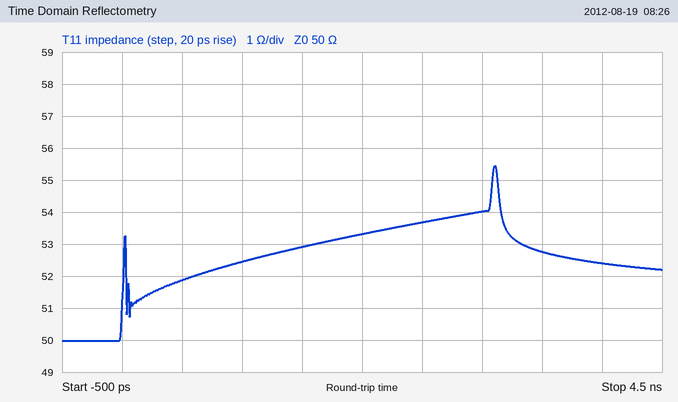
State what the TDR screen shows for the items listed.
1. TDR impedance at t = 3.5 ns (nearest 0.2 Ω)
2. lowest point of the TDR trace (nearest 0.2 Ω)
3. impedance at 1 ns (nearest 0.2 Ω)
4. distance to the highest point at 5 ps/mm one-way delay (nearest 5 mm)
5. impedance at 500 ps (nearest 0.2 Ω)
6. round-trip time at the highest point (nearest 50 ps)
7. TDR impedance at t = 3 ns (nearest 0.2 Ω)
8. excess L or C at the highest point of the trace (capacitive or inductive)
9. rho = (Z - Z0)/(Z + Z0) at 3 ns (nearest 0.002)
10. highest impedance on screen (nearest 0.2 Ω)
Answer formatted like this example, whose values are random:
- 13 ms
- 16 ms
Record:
- 52.8 Ω
- 50.0 Ω
- 52.4 Ω
- 310 mm
- 51.8 Ω
- 3.10 ns
- 54.0 Ω
- inductive
- +0.038
- 55.4 Ω
